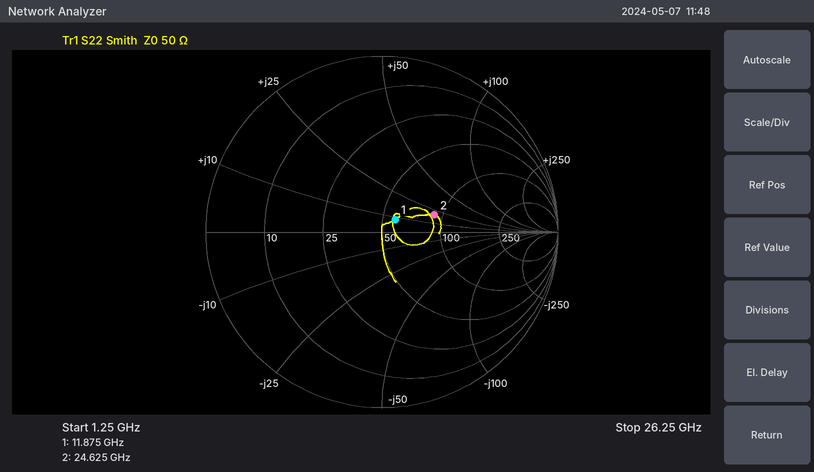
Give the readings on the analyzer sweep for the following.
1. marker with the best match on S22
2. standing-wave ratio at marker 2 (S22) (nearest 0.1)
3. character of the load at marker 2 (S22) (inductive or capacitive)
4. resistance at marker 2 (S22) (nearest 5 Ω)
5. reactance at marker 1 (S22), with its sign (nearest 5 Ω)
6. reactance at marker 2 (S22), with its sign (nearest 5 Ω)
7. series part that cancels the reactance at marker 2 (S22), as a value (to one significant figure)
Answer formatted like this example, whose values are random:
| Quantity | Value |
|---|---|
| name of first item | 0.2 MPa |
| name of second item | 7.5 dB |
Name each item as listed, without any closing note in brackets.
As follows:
| Quantity | Value |
|---|---|
| marker with the best match on S22 | marker 1 |
| standing-wave ratio at marker 2 (S22) | 1.9 |
| character of the load at marker 2 (S22) | inductive |
| resistance at marker 2 (S22) | 90 Ω |
| reactance at marker 1 (S22), with its sign | +10 Ω |
| reactance at marker 2 (S22), with its sign | +20 Ω |
| series part that cancels the reactance at marker 2 (S22), as a value | 300 fF |
